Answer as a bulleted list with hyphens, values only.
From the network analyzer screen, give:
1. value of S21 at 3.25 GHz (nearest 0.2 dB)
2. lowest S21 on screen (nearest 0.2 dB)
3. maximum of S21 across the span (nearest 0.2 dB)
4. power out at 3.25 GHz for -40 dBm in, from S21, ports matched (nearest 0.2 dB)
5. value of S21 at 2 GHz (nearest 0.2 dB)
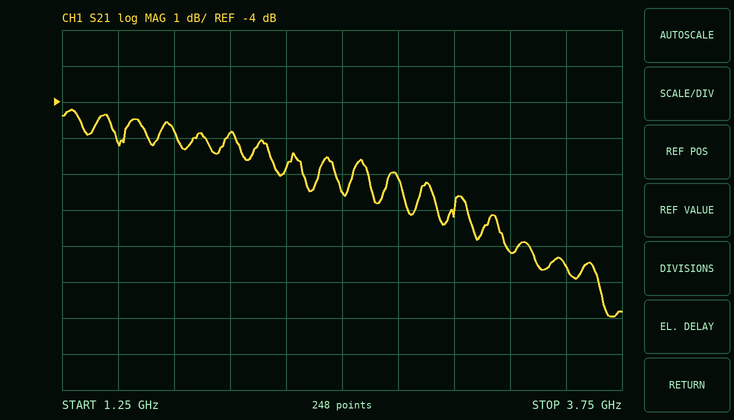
- -8.2 dB
- -10.0 dB
- -4.2 dB
- -48.2 dBm
- -4.8 dB
